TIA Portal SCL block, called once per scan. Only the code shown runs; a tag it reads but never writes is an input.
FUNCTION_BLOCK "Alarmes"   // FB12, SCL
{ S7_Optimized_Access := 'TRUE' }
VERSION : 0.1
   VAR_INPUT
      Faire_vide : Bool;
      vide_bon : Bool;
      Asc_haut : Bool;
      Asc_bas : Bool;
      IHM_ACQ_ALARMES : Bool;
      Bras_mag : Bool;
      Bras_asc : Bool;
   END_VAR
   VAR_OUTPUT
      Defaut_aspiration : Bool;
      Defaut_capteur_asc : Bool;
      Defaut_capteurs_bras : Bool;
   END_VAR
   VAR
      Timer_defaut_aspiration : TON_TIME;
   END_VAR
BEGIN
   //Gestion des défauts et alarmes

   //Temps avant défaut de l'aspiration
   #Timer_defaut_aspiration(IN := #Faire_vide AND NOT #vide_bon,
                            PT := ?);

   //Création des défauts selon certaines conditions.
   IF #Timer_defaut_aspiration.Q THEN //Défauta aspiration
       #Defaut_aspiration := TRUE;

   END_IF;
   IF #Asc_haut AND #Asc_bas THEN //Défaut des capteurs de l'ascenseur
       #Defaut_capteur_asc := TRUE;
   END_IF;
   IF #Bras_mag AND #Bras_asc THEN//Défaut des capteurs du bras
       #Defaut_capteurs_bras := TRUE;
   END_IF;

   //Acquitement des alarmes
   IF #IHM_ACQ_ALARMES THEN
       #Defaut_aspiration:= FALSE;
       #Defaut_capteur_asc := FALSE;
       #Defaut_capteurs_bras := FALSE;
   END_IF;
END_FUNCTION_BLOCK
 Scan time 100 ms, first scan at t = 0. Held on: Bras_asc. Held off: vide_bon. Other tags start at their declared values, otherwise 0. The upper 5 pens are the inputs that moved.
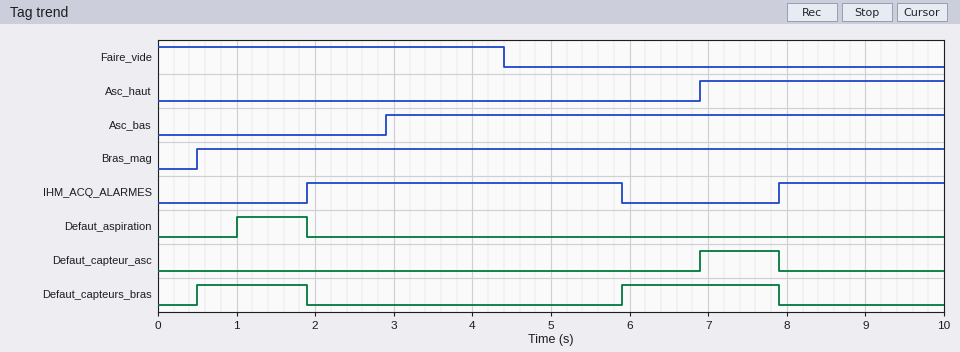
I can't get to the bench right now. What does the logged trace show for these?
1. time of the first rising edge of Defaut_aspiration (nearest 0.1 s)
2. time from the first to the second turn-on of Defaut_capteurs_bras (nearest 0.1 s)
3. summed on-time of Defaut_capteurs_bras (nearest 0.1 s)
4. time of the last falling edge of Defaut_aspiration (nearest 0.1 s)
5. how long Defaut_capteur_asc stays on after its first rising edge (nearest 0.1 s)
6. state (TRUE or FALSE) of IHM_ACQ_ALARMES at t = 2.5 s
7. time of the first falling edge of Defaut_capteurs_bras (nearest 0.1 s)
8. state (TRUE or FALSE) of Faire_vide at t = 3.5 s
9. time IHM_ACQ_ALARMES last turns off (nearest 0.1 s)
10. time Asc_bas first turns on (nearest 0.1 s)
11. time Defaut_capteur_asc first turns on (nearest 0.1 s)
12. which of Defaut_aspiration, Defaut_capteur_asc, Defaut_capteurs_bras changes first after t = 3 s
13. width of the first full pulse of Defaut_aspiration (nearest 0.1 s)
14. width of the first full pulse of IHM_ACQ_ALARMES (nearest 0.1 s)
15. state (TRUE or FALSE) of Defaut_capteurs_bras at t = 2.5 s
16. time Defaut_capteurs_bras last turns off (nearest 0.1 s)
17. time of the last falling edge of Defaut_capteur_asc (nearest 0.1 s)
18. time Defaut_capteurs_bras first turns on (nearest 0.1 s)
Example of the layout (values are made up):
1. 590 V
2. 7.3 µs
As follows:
1. 1.0 s
2. 5.4 s
3. 3.4 s
4. 1.9 s
5. 1.0 s
6. TRUE
7. 1.9 s
8. TRUE
9. 5.9 s
10. 2.9 s
11. 6.9 s
12. Defaut_capteurs_bras
13. 0.9 s
14. 4.0 s
15. FALSE
16. 7.9 s
17. 7.9 s
18. 0.5 s
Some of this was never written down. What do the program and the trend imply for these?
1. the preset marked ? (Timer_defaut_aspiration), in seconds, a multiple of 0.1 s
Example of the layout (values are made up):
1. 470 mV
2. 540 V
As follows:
1. 1.0 s
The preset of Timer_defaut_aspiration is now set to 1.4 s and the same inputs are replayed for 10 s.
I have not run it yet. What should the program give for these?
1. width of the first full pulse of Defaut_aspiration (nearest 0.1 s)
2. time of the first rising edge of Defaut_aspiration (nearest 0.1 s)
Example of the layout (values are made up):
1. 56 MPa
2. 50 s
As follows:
1. 0.5 s
2. 1.4 s
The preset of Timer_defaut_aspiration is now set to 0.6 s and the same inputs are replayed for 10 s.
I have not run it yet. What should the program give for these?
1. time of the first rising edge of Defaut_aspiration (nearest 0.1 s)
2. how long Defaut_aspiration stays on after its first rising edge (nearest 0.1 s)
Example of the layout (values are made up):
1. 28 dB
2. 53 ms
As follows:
1. 0.6 s
2. 1.3 s
